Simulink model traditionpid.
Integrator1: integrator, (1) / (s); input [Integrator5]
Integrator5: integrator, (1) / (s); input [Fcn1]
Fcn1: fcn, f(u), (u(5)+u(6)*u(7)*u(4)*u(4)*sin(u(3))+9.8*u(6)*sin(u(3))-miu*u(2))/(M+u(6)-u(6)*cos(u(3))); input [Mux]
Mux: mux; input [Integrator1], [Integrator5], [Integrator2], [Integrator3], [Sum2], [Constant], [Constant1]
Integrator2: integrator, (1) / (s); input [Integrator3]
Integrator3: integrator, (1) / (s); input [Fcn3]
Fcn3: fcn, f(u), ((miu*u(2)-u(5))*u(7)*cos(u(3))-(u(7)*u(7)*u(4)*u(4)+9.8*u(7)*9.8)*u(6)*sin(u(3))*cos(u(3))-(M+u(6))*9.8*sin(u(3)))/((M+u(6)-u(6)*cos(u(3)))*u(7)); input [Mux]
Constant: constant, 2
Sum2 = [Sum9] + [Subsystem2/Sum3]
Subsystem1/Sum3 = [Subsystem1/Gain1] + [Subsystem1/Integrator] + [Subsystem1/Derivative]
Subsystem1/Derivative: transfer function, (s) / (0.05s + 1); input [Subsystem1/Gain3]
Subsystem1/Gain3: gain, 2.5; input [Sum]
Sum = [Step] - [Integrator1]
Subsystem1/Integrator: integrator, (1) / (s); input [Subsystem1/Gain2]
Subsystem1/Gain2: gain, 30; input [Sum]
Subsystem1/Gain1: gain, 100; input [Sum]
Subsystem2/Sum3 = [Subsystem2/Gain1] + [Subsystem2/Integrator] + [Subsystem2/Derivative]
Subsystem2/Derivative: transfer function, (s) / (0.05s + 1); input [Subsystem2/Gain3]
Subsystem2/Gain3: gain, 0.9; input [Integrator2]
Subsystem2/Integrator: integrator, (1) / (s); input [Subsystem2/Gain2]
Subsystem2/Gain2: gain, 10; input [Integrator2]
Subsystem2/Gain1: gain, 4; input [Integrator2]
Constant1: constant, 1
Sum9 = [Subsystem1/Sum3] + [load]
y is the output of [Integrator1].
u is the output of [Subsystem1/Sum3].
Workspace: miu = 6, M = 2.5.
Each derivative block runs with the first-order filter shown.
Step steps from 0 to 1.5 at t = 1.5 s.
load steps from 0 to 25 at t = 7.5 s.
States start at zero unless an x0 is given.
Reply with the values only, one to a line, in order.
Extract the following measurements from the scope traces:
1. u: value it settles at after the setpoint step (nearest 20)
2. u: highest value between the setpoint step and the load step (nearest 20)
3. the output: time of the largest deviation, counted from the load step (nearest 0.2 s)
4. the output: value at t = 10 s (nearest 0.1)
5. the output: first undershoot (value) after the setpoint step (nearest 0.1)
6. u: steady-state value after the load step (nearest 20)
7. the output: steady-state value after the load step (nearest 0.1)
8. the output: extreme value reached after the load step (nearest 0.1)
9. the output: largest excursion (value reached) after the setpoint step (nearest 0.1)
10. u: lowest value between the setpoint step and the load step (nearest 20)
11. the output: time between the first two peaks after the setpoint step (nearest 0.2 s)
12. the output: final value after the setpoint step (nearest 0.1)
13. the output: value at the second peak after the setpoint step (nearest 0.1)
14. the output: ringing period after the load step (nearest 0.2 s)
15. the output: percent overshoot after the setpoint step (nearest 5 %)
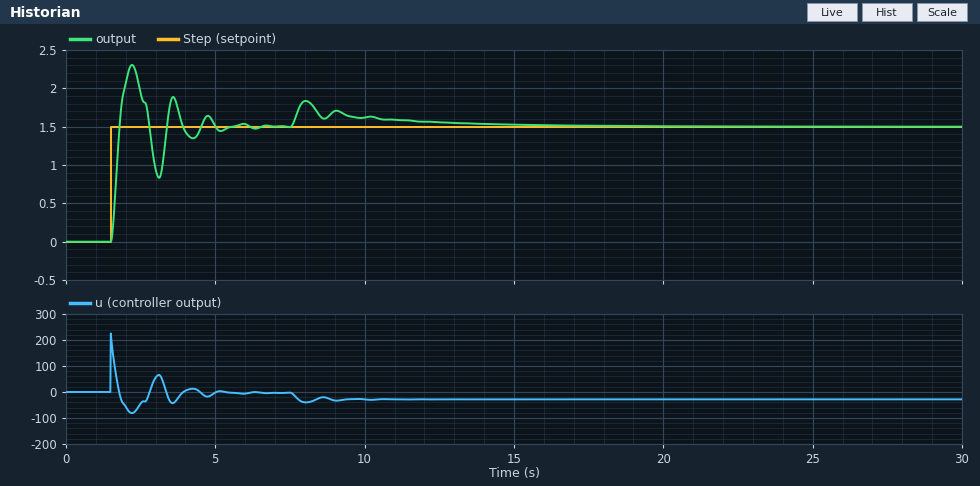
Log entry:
0
220
0.6 s
1.6
0.8
-20
1.5
1.8
2.3
-80
1.4 s
1.5
1.9
1.0 s
55 %
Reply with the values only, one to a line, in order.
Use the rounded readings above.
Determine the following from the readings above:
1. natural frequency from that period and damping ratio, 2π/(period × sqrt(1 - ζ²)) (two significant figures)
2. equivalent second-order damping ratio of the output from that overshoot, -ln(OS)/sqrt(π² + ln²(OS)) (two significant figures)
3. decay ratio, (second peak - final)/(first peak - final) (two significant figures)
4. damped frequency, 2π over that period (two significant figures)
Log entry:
4.6 rad/s
0.19
0.50
4.5 rad/s
